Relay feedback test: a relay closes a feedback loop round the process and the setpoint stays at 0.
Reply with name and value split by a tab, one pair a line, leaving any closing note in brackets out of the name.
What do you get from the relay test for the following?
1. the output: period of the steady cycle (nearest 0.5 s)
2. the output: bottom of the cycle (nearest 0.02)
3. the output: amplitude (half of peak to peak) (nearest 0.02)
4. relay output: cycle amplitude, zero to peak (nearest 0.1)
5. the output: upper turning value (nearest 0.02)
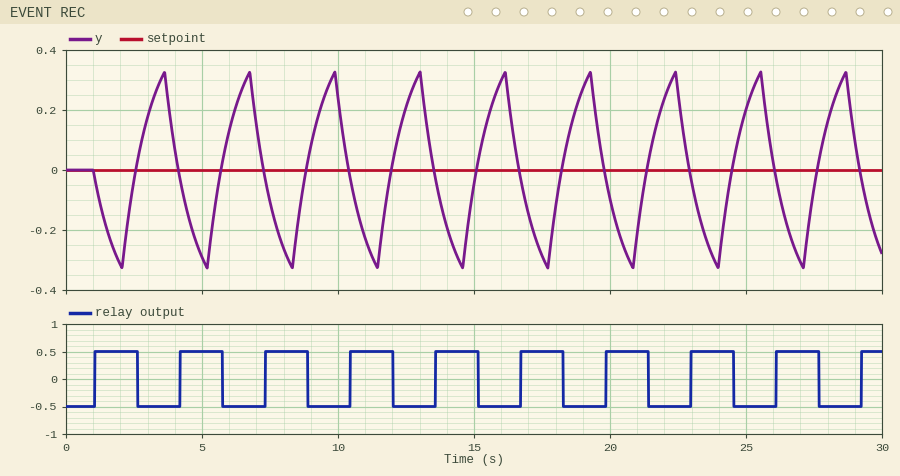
the output: period of the steady cycle	3.0 s
the output: bottom of the cycle	-0.32
the output: amplitude (half of peak to peak)	0.32
relay output: cycle amplitude, zero to peak	0.5
the output: upper turning value	0.32
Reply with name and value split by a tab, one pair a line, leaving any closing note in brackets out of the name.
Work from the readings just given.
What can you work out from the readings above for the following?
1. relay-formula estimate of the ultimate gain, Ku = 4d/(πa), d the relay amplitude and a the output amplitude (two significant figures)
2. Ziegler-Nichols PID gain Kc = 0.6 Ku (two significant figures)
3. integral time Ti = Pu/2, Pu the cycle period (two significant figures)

relay-formula estimate of the ultimate gain, Ku = 4d/(πa), d the relay amplitude and a the output amplitude	2.0
Ziegler-Nichols PID gain Kc = 0.6 Ku	1.2
integral time Ti = Pu/2, Pu the cycle period	1.5 s
